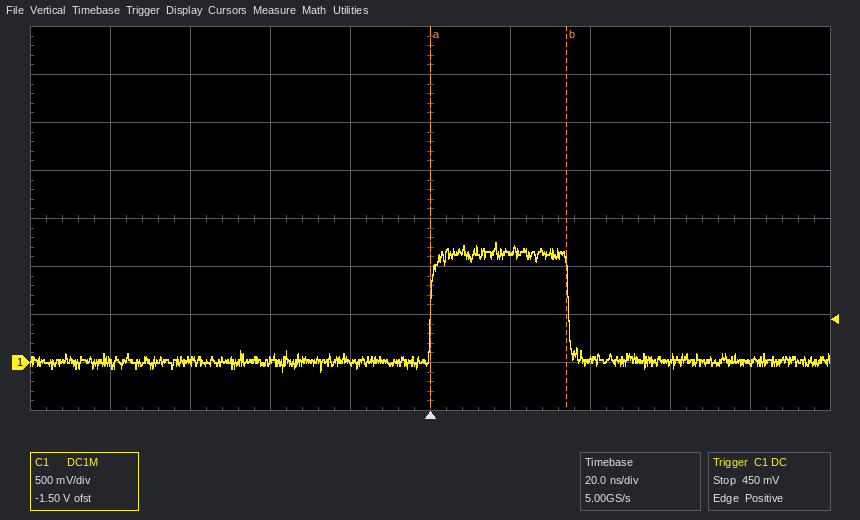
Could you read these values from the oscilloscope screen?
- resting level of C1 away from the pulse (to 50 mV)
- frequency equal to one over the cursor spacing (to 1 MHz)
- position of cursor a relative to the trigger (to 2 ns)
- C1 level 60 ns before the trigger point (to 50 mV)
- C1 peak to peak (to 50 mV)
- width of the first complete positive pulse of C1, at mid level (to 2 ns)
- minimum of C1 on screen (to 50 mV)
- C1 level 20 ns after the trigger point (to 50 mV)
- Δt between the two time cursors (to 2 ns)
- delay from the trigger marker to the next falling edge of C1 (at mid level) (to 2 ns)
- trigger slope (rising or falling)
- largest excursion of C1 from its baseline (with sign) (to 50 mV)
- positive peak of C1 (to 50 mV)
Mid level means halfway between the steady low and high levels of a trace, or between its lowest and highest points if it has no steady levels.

0 mV
29 MHz
0 ns
0 mV
1.35 V
34 ns
-100 mV
1.15 V
34 ns
34 ns
rising
+1.25 V
1.25 V
